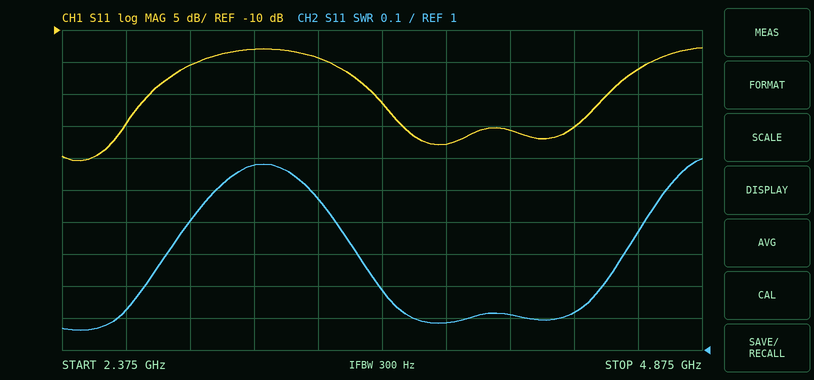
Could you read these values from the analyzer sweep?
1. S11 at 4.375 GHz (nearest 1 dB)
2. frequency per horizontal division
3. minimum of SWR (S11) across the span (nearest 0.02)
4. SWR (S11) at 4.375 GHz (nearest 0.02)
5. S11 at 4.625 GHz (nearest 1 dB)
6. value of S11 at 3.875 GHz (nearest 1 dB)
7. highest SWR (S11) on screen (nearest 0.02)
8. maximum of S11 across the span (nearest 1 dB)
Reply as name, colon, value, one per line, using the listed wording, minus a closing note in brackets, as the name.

S11 at 4.375 GHz: -25 dB
frequency per horizontal division: 250 MHz
minimum of SWR (S11) across the span: 1.06
SWR (S11) at 4.375 GHz: 1.12
S11 at 4.625 GHz: -16 dB
value of S11 at 3.875 GHz: -28 dB
highest SWR (S11) on screen: 1.60
maximum of S11 across the span: -13 dB
